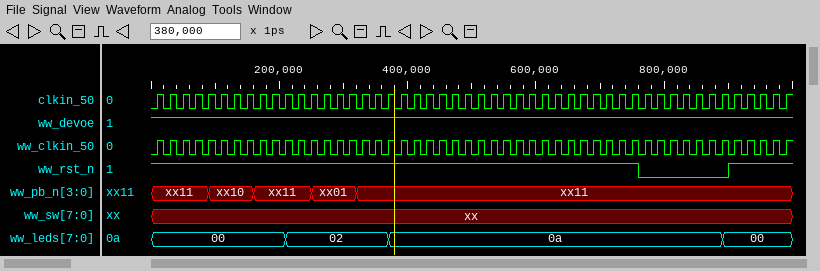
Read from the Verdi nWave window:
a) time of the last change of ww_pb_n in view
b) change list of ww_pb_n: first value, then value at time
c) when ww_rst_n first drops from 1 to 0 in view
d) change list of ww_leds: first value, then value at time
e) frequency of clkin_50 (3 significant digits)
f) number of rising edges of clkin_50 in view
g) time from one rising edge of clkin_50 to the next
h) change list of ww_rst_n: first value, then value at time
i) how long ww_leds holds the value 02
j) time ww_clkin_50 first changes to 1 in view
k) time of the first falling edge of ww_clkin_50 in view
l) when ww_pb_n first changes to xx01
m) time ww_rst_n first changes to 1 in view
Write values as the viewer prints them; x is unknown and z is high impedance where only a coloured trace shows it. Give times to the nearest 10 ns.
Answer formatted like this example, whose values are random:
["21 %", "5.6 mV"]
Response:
["320 ns", "xx11, xx10 at 90 ns, xx11 at 160 ns, xx01 at 250 ns, xx11 at 320 ns", "760 ns", "00, 02 at 210 ns, 0a at 370 ns, 00 at 890 ns", "50.0 MHz", "50", "20 ns", "1, 0 at 760 ns, 1 at 900 ns", "160 ns", "10 ns", "20 ns", "250 ns", "900 ns"]
